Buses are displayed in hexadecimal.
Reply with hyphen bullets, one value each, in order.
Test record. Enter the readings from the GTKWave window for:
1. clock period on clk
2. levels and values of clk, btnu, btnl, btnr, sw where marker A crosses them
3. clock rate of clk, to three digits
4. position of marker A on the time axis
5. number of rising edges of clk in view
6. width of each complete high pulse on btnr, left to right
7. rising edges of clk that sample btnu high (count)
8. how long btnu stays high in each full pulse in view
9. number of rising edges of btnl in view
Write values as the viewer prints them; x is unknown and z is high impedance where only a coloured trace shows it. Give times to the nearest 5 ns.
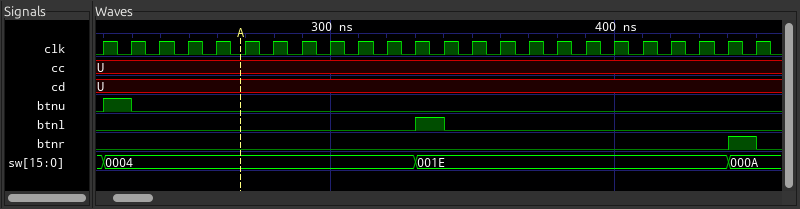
- 10 ns
- clk=0, btnu=0, btnl=0, btnr=0, sw=0004
- 100 MHz
- 270 ns
- 24
- 10 ns
- 1
- 10 ns
- 1
